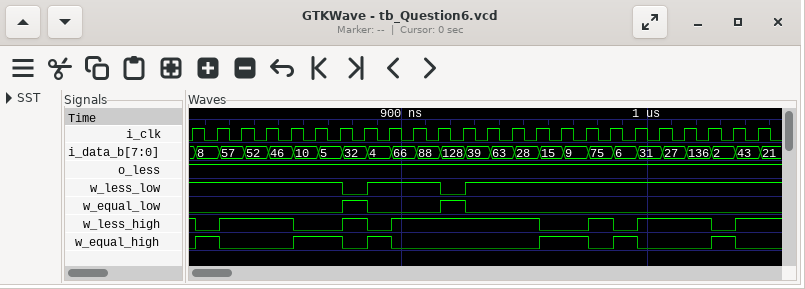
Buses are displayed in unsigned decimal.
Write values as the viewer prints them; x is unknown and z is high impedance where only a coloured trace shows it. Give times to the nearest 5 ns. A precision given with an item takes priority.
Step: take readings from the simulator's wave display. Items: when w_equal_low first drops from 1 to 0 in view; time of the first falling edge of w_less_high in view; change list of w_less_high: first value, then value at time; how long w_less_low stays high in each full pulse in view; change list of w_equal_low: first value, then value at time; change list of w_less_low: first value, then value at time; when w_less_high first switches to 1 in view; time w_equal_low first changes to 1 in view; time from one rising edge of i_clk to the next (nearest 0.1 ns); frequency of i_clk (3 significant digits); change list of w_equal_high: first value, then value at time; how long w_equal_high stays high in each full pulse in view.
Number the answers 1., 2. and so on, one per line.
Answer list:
1. 885 ns
2. 815 ns
3. 1, 0 at 815 ns, 1 at 825 ns, 0 at 855 ns, 1 at 875 ns, 0 at 885 ns, 1 at 895 ns, 0 at 955 ns, 1 at 975 ns, 0 at 985 ns, 1 at 995 ns, 0 at 1025 ns, 1 at 1035 ns
4. 30 ns
5. 0, 1 at 875 ns, 0 at 885 ns, 1 at 915 ns, 0 at 925 ns
6. 1, 0 at 875 ns, 1 at 885 ns, 0 at 915 ns, 1 at 925 ns
7. 825 ns
8. 875 ns
9. 10 ns
10. 100 MHz
11. 0, 1 at 815 ns, 0 at 825 ns, 1 at 855 ns, 0 at 875 ns, 1 at 885 ns, 0 at 895 ns, 1 at 955 ns, 0 at 975 ns, 1 at 985 ns, 0 at 995 ns, 1 at 1025 ns, 0 at 1035 ns
12. 10 ns, 20 ns, 10 ns, 20 ns, 10 ns, 10 ns
